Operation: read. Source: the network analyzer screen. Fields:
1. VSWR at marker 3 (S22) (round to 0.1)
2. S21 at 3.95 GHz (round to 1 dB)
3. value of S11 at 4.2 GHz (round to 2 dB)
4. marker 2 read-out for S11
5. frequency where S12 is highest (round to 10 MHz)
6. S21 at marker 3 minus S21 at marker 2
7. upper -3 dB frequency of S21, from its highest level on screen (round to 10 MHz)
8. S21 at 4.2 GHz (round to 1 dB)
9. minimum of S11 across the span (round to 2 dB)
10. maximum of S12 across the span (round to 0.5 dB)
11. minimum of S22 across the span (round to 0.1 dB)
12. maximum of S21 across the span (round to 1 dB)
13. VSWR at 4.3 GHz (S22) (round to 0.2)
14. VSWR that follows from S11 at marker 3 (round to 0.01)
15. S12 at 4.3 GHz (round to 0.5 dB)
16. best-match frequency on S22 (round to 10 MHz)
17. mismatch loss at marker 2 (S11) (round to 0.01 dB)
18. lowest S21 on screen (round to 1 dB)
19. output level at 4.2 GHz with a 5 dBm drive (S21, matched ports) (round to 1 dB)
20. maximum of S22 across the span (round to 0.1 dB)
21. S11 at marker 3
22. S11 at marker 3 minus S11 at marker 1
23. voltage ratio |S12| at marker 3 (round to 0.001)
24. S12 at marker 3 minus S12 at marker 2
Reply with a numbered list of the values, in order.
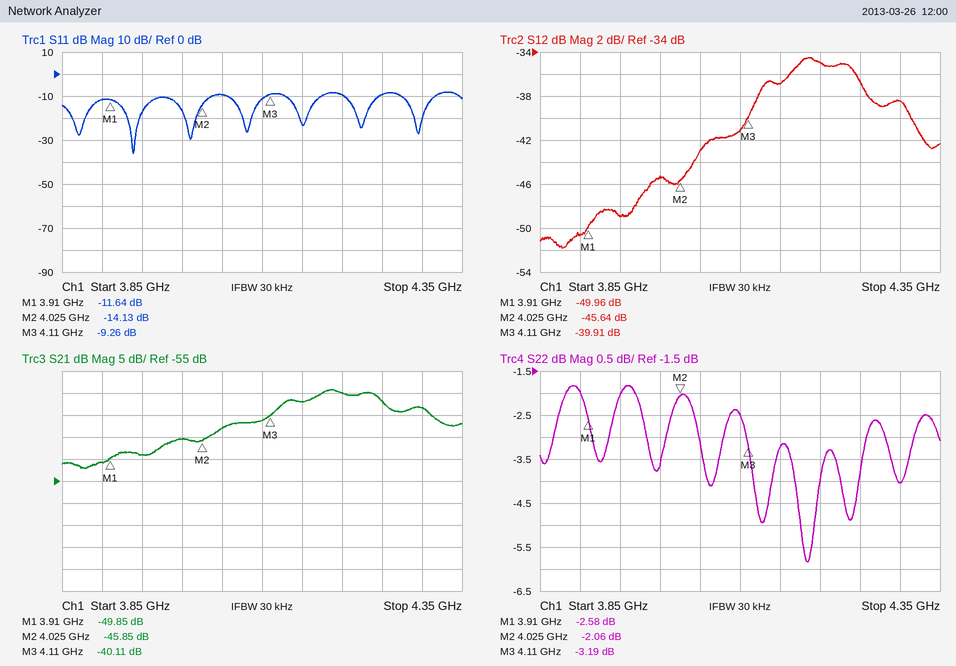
1. 5.5
2. -49 dB
3. -10 dB
4. -14.13 dB
5. 4.19 GHz
6. 5.74 dB
7. 4.25 GHz
8. -35 dB
9. -36 dB
10. -34.5 dB
11. -5.8 dB
12. -34 dB
13. 4.4
14. 2.05
15. -38.5 dB
16. 4.18 GHz
17. 0.17 dB
18. -52 dB
19. -30 dBm
20. -1.8 dB
21. -9.26 dB
22. 2.38 dB
23. 0.010
24. 5.73 dB
